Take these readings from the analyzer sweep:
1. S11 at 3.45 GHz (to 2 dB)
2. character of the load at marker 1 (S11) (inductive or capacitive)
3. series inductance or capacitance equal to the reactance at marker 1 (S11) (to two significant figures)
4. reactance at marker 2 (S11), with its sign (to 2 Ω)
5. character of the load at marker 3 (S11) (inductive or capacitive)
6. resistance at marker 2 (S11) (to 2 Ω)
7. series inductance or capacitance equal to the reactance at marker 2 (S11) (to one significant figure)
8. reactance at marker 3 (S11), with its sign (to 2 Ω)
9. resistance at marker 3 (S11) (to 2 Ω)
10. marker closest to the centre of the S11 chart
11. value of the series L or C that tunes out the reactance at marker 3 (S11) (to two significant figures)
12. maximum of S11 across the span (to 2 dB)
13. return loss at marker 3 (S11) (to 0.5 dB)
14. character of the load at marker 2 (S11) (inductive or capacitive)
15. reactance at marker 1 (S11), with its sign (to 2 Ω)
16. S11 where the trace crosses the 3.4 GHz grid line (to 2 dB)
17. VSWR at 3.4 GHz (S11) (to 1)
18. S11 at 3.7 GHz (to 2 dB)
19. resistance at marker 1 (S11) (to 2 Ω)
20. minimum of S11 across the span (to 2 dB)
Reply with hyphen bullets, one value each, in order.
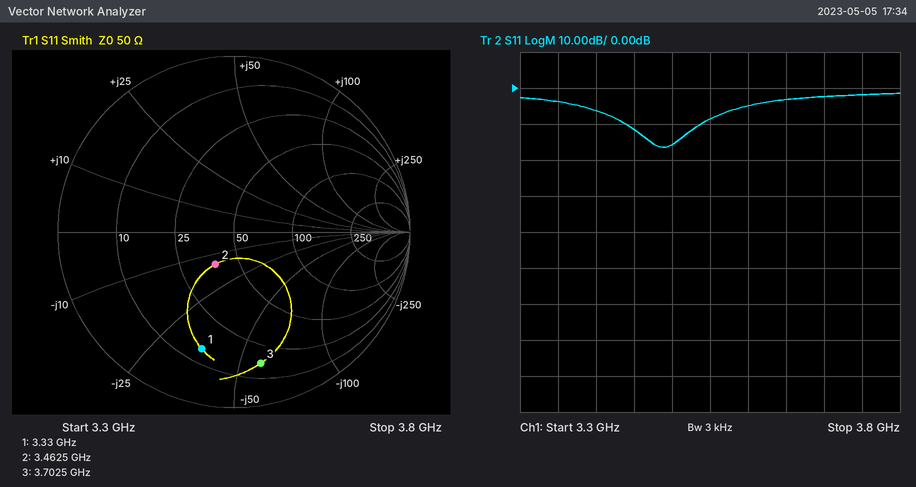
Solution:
- -12 dB
- capacitive
- 1.3 pF
- -14 Ω
- capacitive
- 38 Ω
- 3 pF
- -58 Ω
- 16 Ω
- marker 2
- 2.5 nH
- -2 dB
- 2.5 dB
- capacitive
- -36 Ω
- -6 dB
- 3
- -2 dB
- 14 Ω
- -16 dB
